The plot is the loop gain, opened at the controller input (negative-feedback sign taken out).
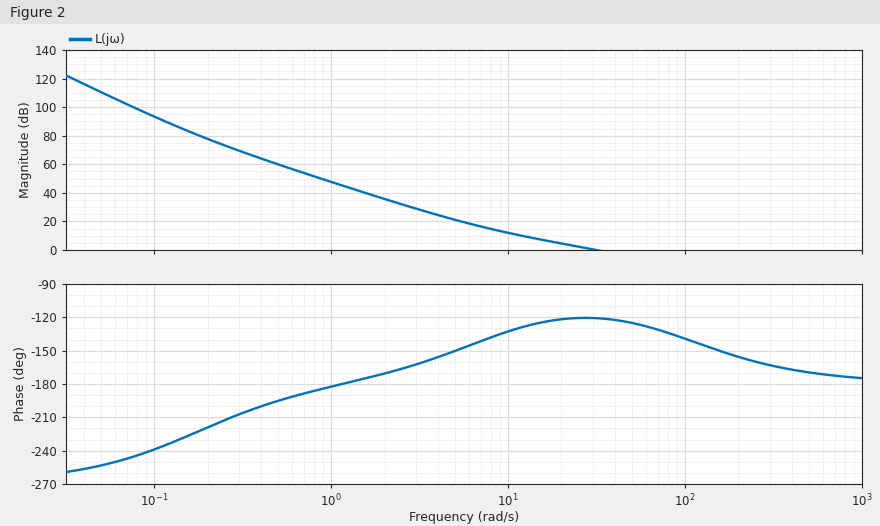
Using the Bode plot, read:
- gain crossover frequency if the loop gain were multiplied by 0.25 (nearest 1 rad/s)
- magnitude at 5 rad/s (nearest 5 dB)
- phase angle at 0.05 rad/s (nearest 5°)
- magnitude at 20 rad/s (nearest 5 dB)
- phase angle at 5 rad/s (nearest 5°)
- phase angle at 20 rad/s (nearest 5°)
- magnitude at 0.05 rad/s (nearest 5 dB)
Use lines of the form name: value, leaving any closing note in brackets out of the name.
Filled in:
gain crossover frequency if the loop gain were multiplied by 0.25: 10 rad/s
magnitude at 5 rad/s: 20 dB
phase angle at 0.05 rad/s: -255°
magnitude at 20 rad/s: 5 dB
phase angle at 5 rad/s: -150°
phase angle at 20 rad/s: -120°
magnitude at 0.05 rad/s: 110 dB
